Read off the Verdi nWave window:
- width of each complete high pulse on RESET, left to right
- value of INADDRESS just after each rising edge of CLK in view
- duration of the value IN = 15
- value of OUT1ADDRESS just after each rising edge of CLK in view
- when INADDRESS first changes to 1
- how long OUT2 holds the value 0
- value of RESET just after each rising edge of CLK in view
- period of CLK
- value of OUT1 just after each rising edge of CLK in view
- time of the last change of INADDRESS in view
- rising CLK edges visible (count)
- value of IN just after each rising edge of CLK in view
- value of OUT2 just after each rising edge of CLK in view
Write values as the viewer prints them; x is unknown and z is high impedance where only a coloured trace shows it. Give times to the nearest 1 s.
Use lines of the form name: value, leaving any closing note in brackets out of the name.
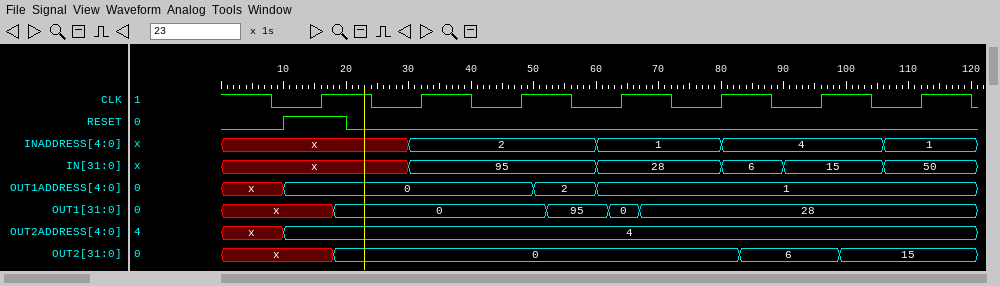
width of each complete high pulse on RESET, left to right: 10 s
value of INADDRESS just after each rising edge of CLK in view: x, 2, 2, 1, 4, 4, 1
duration of the value IN = 15: 16 s
value of OUT1ADDRESS just after each rising edge of CLK in view: 0, 0, 0, 1, 1, 1, 1
when INADDRESS first changes to 1: 60 s
how long OUT2 holds the value 0: 65 s
value of RESET just after each rising edge of CLK in view: 1 0 0 0 0 0 0
period of CLK: 16 s
value of OUT1 just after each rising edge of CLK in view: x, 0, 0, 0, 28, 28, 28
time of the last change of INADDRESS in view: 106 s
rising CLK edges visible: 7
value of IN just after each rising edge of CLK in view: x, 95, 95, 28, 6, 15, 50
value of OUT2 just after each rising edge of CLK in view: x, 0, 0, 0, 0, 6, 15
